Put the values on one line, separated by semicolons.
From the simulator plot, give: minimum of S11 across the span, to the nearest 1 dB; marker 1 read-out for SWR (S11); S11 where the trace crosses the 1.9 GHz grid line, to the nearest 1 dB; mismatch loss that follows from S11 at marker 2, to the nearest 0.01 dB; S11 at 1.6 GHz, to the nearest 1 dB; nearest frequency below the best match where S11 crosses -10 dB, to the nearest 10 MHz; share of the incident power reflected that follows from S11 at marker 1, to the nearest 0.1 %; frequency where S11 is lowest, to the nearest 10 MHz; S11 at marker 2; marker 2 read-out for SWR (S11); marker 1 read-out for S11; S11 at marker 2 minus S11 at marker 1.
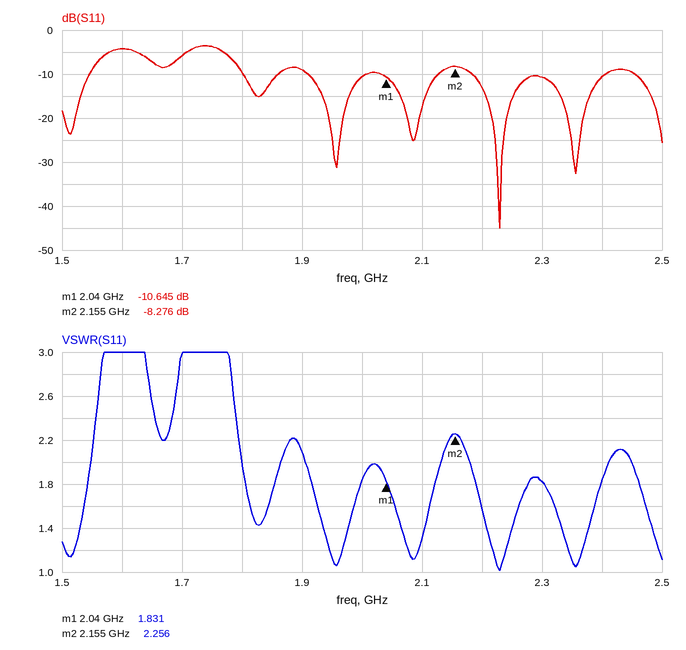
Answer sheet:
-45 dB; 1.831; -9 dB; 0.70 dB; -4 dB; 2.18 GHz; 8.6 %; 2.23 GHz; -8.276 dB; 2.256; -10.645 dB; 2.369 dB
